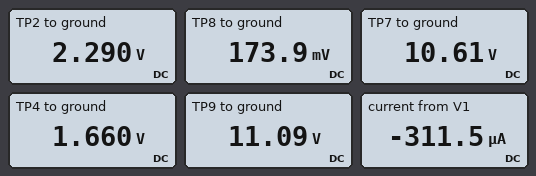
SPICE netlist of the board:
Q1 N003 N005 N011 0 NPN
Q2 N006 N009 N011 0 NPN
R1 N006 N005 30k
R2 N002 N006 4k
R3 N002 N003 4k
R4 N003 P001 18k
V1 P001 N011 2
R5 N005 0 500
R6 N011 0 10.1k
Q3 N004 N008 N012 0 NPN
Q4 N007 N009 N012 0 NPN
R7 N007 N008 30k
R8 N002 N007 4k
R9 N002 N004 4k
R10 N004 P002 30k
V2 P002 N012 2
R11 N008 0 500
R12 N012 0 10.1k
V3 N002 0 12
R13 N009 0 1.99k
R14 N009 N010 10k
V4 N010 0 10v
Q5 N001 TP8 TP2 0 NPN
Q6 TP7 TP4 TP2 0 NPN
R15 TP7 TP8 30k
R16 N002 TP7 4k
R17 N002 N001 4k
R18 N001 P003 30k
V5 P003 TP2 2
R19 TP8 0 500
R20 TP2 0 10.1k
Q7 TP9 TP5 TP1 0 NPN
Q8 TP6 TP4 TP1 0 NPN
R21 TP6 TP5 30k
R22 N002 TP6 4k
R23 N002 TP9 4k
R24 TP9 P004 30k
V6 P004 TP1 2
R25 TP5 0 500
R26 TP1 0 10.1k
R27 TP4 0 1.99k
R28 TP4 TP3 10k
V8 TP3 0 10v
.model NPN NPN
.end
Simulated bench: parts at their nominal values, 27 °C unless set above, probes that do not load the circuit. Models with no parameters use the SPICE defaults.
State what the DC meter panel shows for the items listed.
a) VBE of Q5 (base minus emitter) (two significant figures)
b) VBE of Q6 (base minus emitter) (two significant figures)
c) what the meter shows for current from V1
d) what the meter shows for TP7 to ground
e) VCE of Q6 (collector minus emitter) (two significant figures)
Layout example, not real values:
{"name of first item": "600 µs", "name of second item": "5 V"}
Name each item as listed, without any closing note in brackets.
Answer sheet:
{"VBE of Q5 (base minus emitter)": "-2.1 V", "VBE of Q6 (base minus emitter)": "-630 mV", "what the meter shows for current from V1": "-311.5 µA", "what the meter shows for TP7 to ground": "10.61 V", "VCE of Q6 (collector minus emitter)": "8.3 V"}
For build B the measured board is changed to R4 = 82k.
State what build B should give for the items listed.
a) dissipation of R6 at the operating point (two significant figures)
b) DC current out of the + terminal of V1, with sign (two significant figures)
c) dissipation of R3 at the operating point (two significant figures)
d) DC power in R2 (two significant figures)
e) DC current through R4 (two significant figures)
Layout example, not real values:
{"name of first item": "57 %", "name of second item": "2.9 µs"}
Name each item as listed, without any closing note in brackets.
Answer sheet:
{"dissipation of R6 at the operating point": "110 µW", "DC current out of the + terminal of V1, with sign": "-100 µA", "dissipation of R3 at the operating point": "43 µW", "DC power in R2": "490 µW", "DC current through R4": "100 µA"}
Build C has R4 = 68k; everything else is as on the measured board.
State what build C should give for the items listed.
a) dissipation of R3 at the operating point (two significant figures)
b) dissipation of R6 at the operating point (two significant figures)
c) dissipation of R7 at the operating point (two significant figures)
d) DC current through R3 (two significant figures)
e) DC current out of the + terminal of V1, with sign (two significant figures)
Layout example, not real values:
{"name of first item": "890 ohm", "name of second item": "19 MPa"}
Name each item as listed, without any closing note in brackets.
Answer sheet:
{"dissipation of R3 at the operating point": "59 µW", "dissipation of R6 at the operating point": "150 µW", "dissipation of R7 at the operating point": "3.6 mW", "DC current through R3": "120 µA", "DC current out of the + terminal of V1, with sign": "-120 µA"}
